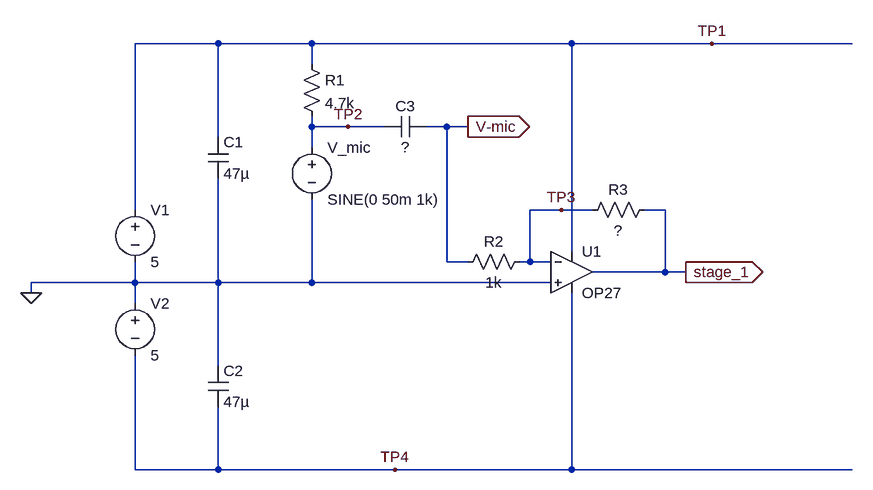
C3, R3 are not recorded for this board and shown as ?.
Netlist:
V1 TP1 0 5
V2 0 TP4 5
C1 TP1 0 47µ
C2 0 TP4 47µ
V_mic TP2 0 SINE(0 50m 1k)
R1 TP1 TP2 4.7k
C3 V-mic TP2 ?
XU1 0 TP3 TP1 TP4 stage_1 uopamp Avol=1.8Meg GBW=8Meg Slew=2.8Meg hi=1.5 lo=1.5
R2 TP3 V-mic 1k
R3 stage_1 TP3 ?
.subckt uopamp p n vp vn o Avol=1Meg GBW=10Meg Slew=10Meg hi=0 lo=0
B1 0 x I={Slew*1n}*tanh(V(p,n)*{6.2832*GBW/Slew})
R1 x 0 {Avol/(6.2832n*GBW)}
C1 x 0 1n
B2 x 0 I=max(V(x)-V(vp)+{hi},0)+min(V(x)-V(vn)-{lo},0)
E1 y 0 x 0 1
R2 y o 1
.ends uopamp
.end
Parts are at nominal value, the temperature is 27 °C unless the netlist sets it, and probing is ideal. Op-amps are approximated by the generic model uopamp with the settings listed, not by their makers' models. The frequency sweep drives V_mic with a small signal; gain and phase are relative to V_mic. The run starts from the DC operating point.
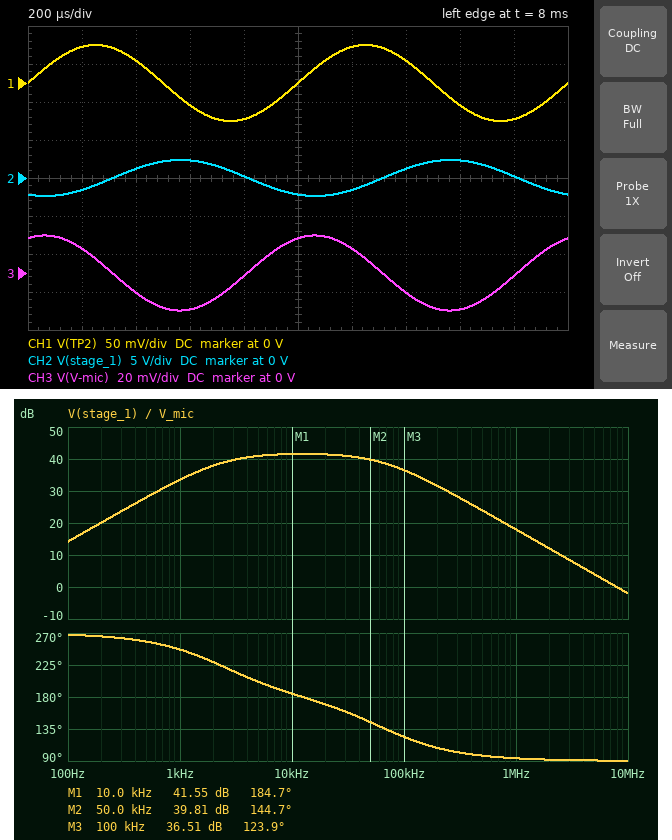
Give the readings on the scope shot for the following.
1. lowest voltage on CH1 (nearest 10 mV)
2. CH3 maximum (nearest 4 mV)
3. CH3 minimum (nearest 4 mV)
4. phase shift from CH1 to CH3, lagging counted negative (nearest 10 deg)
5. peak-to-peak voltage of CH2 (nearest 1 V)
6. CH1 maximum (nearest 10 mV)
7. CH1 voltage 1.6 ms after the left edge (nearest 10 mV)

-50 mV
20 mV
-20 mV
70 deg
5 V
50 mV
-30 mV
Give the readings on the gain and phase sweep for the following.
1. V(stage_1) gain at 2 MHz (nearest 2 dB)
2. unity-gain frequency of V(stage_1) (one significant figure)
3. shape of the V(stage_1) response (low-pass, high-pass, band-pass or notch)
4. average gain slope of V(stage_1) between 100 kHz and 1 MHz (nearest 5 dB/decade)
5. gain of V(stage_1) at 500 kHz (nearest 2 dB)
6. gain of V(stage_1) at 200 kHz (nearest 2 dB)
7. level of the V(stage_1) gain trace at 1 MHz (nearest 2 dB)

12 dB
8 MHz
band-pass
-20 dB/decade
24 dB
32 dB
18 dB
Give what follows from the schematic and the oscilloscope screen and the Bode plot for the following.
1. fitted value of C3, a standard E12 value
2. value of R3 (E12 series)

68 nF
120 kΩ
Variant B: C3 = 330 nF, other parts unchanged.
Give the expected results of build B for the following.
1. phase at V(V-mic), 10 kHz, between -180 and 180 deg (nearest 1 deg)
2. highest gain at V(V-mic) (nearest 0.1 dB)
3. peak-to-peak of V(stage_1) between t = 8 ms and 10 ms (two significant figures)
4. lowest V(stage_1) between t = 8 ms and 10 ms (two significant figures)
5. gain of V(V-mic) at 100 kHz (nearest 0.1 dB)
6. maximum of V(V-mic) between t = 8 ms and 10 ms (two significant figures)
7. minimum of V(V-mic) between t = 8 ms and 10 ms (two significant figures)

3 deg
0.1 dB
7.0 V
-3.5 V
0 dB
47 mV
-47 mV
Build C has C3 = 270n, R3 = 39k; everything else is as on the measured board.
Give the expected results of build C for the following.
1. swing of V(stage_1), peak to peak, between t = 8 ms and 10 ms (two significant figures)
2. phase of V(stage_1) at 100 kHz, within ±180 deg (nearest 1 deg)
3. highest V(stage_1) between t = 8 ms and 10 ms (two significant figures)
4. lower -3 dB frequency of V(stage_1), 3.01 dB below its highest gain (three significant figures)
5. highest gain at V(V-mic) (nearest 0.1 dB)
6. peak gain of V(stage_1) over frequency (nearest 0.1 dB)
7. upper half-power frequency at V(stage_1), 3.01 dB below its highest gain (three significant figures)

3.4 V
154 deg
1.7 V
588 Hz
0 dB
31.8 dB
201 kHz
